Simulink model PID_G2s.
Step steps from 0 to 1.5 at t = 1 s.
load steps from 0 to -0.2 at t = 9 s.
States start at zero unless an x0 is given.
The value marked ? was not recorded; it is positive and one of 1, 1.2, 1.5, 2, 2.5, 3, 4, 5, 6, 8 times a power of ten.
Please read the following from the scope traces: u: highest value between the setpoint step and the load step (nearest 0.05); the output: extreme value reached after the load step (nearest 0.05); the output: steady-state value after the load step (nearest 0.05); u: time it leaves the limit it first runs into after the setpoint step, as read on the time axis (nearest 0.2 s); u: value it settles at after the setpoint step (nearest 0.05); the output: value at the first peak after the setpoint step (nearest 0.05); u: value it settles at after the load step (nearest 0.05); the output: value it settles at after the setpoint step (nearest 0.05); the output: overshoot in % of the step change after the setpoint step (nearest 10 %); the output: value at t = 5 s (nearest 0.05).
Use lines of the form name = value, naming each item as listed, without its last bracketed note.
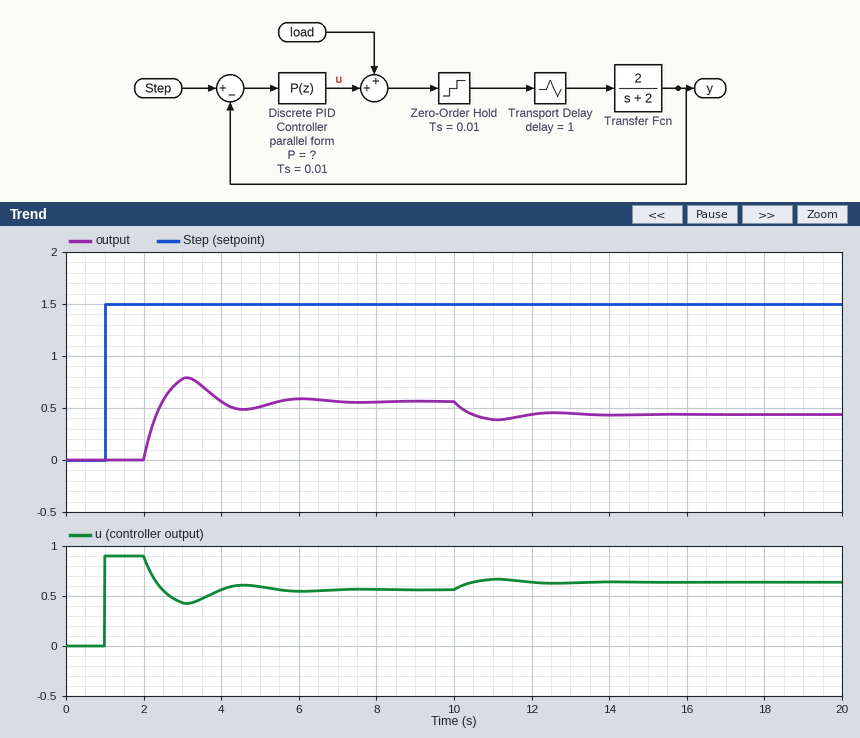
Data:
u: highest value between the setpoint step and the load step = 0.90
the output: extreme value reached after the load step = 0.40
the output: steady-state value after the load step = 0.45
u: time it leaves the limit it first runs into after the setpoint step, as read on the time axis = 2.0 s
u: value it settles at after the setpoint step = 0.55
the output: value at the first peak after the setpoint step = 0.80
u: value it settles at after the load step = 0.65
the output: value it settles at after the setpoint step = 0.55
the output: overshoot in % of the step change after the setpoint step = 40 %
the output: value at t = 5 s = 0.50
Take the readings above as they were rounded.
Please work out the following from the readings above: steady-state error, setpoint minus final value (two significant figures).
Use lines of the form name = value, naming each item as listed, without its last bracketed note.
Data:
steady-state error, setpoint minus final value = 0.95
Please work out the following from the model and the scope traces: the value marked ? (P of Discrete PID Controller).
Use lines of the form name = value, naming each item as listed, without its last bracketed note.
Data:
the value marked ? = 0.6
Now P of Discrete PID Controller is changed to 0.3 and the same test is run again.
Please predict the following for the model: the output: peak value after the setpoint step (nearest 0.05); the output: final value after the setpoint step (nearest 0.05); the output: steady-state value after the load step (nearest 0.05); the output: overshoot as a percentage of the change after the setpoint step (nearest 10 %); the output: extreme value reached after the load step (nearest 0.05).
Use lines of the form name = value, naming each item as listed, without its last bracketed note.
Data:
the output: peak value after the setpoint step = 0.40
the output: final value after the setpoint step = 0.35
the output: steady-state value after the load step = 0.20
the output: overshoot as a percentage of the change after the setpoint step = 20 %
the output: extreme value reached after the load step = 0.15
